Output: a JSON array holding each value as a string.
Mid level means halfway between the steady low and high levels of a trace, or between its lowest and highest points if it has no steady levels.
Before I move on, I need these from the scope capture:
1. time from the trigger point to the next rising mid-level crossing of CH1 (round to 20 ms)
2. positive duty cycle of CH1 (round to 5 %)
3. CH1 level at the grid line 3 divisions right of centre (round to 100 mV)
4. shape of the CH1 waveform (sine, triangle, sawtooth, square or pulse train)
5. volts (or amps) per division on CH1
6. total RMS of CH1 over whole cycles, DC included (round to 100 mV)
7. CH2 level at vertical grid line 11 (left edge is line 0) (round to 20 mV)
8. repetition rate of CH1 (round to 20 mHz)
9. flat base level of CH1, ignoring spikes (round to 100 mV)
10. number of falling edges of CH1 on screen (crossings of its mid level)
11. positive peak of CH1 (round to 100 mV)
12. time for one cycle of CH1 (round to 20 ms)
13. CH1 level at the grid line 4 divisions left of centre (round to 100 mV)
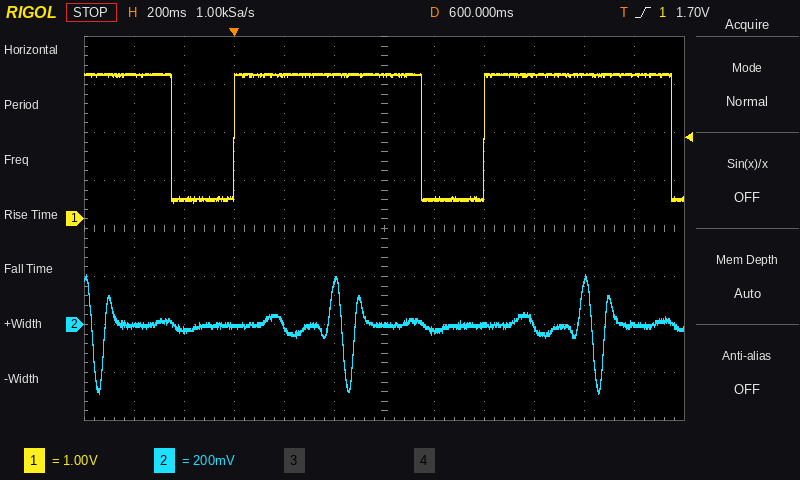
["1.00 s", "75 %", "3.0 V", "pulse train", "1 V", "2.6 V", "0 mV", "1.00 Hz", "400 mV", "3", "3.0 V", "1.00 s", "400 mV"]
